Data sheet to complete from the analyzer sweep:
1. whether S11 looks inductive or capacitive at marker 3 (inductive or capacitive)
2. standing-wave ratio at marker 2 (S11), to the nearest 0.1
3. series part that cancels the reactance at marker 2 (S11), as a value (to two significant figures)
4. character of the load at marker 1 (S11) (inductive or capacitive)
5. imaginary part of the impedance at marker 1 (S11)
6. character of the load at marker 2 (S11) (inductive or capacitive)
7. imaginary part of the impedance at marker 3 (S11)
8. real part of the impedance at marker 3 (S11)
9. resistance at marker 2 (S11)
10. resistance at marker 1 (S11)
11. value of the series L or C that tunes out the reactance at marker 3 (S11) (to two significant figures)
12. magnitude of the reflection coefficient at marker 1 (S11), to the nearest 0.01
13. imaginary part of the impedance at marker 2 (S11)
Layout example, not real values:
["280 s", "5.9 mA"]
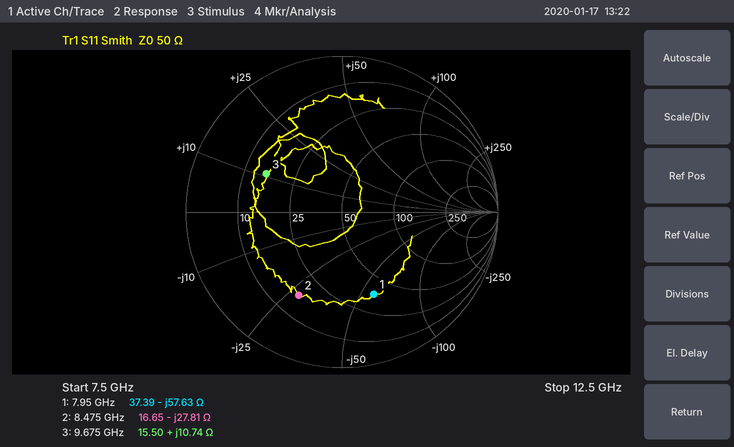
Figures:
["inductive", "4.0", "520 pH", "capacitive", "-57.63 Ω", "capacitive", "+10.74 Ω", "15.50 Ω", "16.65 Ω", "37.39 Ω", "1.5 pF", "0.56", "-27.81 Ω"]
